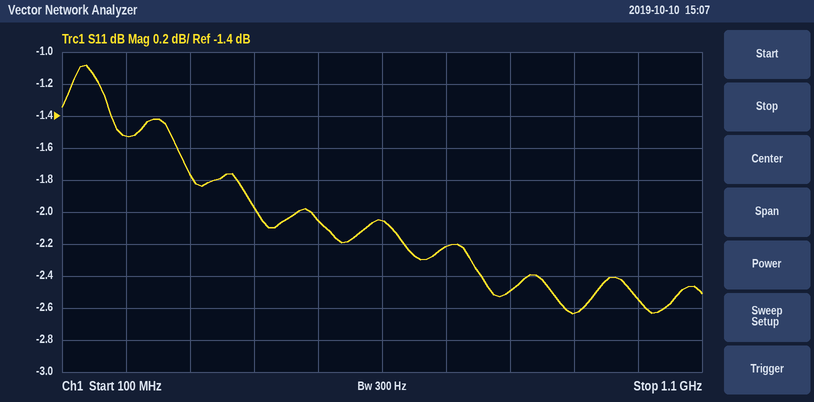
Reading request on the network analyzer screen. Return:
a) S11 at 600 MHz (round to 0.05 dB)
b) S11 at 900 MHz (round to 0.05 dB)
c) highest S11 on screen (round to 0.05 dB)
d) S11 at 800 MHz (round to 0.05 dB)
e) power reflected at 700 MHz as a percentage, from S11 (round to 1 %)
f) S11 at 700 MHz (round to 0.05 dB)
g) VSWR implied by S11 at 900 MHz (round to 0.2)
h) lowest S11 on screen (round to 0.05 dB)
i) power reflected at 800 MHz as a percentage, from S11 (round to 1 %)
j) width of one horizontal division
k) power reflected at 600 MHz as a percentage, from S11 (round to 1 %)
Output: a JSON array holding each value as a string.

["-2.05 dB", "-2.65 dB", "-1.10 dB", "-2.50 dB", "60 %", "-2.20 dB", "6.6", "-2.65 dB", "56 %", "100 MHz", "62 %"]
